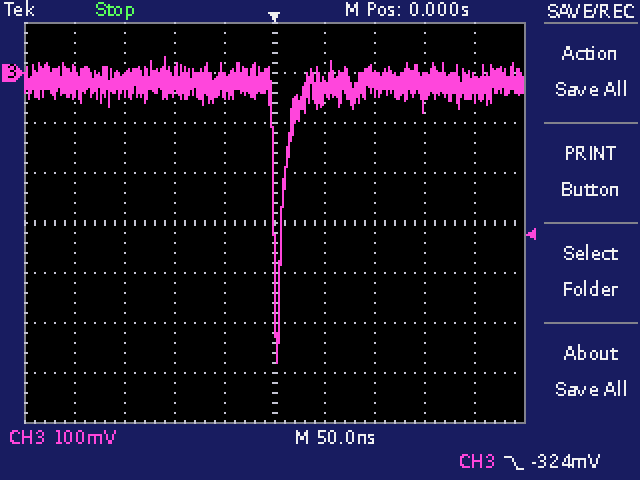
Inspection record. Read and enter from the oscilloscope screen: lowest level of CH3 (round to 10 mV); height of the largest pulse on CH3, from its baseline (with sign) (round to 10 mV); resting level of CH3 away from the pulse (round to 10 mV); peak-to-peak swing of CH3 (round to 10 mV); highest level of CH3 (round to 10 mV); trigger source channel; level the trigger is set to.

-580 mV
-560 mV
-20 mV
610 mV
30 mV
CH3
-324 mV
